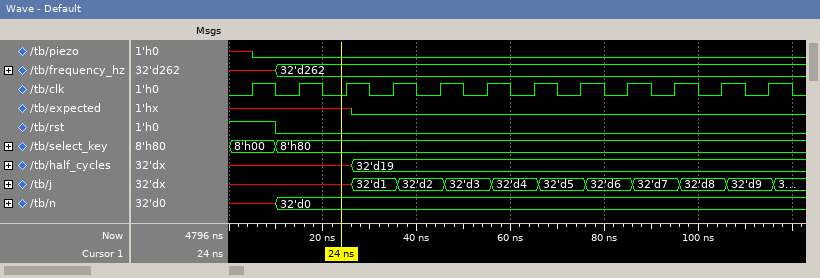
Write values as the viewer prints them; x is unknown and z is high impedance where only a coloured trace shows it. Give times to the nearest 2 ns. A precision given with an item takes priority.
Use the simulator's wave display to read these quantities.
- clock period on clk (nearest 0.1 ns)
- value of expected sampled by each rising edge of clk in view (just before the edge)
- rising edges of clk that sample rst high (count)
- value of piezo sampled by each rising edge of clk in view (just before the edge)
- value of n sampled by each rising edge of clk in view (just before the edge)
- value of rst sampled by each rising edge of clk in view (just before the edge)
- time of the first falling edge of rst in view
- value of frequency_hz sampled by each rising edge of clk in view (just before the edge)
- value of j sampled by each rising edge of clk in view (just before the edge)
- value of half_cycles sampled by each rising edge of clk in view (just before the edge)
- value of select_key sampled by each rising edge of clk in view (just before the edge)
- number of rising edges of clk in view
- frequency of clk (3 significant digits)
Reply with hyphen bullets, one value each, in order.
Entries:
- 10 ns
- x x x 0 0 0 0 0 0 0 0 0
- 1
- x 0 0 0 0 0 0 0 0 0 0 0
- x, 32'd0, 32'd0, 32'd0, 32'd0, 32'd0, 32'd0, 32'd0, 32'd0, 32'd0, 32'd0, 32'd0
- 1 0 0 0 0 0 0 0 0 0 0 0
- 10 ns
- x, 32'd262, 32'd262, 32'd262, 32'd262, 32'd262, 32'd262, 32'd262, 32'd262, 32'd262, 32'd262, 32'd262
- x, x, x, 32'd1, 32'd2, 32'd3, 32'd4, 32'd5, 32'd6, 32'd7, 32'd8, 32'd9
- x, x, x, 32'd19, 32'd19, 32'd19, 32'd19, 32'd19, 32'd19, 32'd19, 32'd19, 32'd19
- 8'h00, 8'h80, 8'h80, 8'h80, 8'h80, 8'h80, 8'h80, 8'h80, 8'h80, 8'h80, 8'h80, 8'h80
- 12
- 100 MHz
